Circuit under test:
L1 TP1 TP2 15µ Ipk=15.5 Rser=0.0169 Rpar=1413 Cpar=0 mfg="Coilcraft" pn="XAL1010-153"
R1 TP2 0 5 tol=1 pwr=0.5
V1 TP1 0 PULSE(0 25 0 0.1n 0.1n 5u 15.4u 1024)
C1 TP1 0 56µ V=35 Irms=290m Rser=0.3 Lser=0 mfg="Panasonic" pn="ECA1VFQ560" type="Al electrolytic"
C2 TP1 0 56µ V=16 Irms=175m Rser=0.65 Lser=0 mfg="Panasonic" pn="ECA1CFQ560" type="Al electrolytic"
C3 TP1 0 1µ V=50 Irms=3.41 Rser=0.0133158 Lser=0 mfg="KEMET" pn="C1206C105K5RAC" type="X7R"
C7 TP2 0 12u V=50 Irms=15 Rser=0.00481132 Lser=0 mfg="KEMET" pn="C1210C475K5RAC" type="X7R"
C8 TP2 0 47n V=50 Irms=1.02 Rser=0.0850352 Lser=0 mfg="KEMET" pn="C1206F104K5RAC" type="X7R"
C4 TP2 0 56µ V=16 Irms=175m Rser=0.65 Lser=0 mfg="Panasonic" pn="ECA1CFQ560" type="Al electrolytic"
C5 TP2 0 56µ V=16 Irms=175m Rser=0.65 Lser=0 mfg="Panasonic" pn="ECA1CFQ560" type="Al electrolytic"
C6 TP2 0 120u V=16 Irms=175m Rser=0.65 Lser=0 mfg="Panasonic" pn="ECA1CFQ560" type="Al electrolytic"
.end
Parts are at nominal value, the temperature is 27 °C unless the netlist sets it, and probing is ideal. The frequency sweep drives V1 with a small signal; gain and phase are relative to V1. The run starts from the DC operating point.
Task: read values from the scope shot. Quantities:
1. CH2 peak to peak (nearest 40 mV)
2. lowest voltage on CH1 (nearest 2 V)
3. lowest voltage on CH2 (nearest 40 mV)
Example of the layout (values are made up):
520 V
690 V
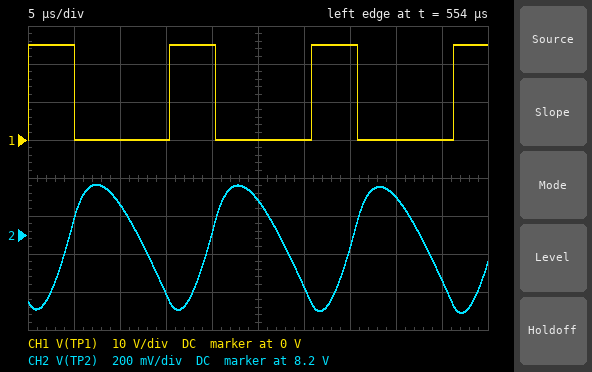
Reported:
680 mV
0 V
7.80 V
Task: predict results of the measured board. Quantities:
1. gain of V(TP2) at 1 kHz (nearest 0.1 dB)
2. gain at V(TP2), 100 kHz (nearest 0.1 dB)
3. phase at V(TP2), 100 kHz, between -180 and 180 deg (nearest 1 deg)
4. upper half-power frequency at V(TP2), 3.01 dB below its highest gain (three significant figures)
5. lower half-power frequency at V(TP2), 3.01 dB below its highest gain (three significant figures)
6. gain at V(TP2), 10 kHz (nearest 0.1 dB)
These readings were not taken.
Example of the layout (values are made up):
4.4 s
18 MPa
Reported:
1.0 dB
-38.7 dB
-146 deg
3.66 kHz
486 Hz
-12.4 dB
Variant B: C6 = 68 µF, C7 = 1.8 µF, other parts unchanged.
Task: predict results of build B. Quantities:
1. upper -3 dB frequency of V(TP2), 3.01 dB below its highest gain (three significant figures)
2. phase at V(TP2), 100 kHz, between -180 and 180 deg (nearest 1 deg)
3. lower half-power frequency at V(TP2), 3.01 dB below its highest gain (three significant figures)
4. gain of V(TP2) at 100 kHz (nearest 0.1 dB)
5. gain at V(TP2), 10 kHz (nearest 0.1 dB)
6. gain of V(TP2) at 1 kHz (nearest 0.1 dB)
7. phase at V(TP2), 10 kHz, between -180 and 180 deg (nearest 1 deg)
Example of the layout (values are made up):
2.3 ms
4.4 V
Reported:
3.87 kHz
-104 deg
906 Hz
-33.4 dB
-12.0 dB
0.8 dB
-98 deg
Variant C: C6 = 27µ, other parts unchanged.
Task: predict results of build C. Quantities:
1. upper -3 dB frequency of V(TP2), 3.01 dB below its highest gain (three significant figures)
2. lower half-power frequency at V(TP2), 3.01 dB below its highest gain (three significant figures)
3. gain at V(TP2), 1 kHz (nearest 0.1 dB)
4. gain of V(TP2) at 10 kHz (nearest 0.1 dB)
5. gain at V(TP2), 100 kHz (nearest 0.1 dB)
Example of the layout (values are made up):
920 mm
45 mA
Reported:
4.26 kHz
1.47 kHz
0.7 dB
-11.5 dB
-38.8 dB
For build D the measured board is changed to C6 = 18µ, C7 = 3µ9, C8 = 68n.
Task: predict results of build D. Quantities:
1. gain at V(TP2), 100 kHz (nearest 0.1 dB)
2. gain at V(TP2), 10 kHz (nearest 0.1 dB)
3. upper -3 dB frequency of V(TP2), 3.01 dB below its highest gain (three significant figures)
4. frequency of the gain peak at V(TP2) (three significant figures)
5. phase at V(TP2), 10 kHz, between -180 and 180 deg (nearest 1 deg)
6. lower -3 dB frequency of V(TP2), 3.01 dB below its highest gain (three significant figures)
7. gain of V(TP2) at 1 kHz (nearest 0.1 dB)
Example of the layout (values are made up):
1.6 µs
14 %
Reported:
-34.3 dB
-10.4 dB
4.58 kHz
3.14 kHz
-106 deg
1.26 kHz
0.6 dB
